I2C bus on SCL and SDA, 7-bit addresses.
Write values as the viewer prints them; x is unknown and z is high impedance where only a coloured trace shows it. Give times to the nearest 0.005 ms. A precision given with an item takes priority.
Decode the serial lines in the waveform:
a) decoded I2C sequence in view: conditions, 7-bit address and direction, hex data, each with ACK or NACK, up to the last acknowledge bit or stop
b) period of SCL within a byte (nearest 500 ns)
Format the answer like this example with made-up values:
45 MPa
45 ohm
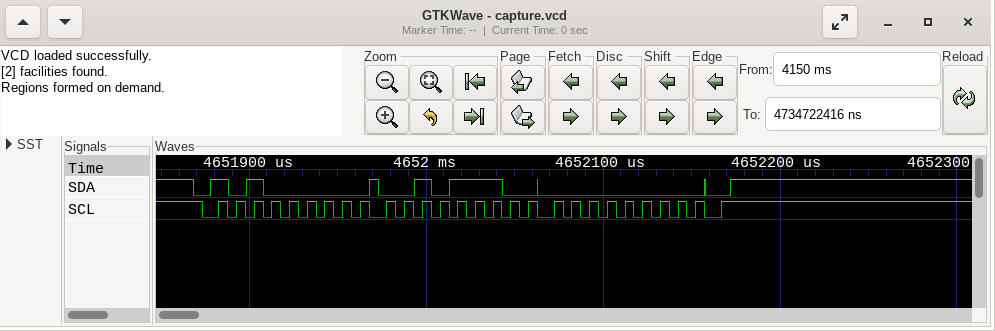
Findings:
start, address 50 write ACK, 2E ACK, 00 ACK, stop
10000 ns
